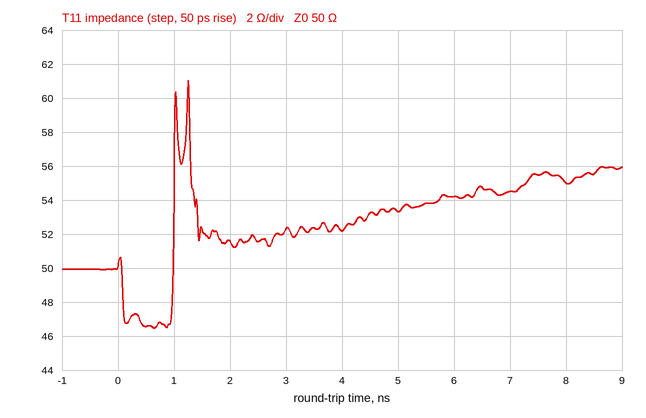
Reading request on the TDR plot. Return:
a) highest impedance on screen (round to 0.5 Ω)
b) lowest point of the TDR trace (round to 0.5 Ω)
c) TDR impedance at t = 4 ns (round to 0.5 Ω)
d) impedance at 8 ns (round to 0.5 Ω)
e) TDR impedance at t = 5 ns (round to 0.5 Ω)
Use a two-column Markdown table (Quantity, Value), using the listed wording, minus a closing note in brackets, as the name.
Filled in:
| Quantity | Value |
|---|---|
| highest impedance on screen | 61.0 Ω |
| lowest point of the TDR trace | 46.5 Ω |
| TDR impedance at t = 4 ns | 52.0 Ω |
| impedance at 8 ns | 55.0 Ω |
| TDR impedance at t = 5 ns | 53.5 Ω |
